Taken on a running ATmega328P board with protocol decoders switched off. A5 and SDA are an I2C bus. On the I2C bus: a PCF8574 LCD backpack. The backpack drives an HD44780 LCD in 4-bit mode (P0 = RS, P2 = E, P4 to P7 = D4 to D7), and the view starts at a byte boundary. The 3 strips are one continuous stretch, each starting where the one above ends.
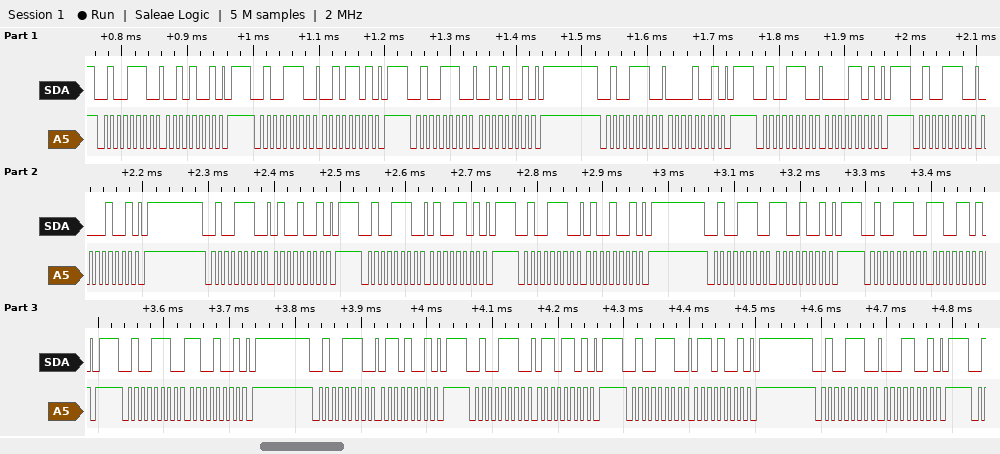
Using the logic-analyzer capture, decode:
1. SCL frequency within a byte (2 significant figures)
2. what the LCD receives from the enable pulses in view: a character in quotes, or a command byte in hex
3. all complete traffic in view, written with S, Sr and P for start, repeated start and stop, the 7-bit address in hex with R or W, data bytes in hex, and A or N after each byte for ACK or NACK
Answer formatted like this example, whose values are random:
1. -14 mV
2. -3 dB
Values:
1. 100 kHz
2. ' ' 'L'
3. S 27W A 29 A P S 27W A 2D A P S 27W A 29 A P S 27W A 09 A P S 27W A 0D A P S 27W A 09 A P S 27W A 49 A P S 27W A 4D A P S 27W A 49 A P S 27W A C9 A P S 27W A CD A P S 27W A C9 A P S 27W A 69 A P S 27W A 6D A P S 27W A 69 A P S 27W A 19 A P
